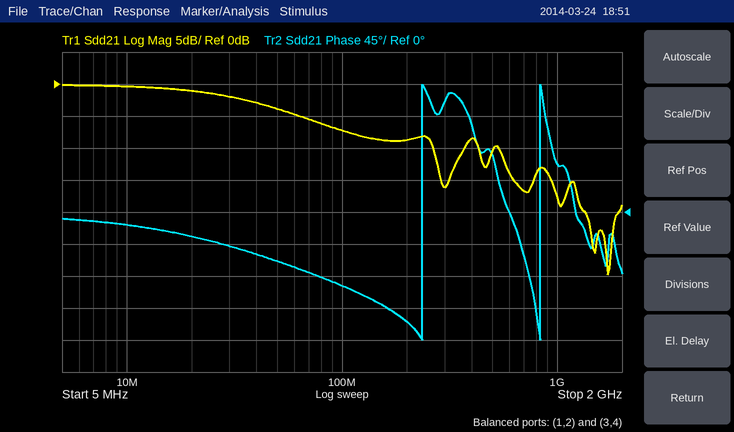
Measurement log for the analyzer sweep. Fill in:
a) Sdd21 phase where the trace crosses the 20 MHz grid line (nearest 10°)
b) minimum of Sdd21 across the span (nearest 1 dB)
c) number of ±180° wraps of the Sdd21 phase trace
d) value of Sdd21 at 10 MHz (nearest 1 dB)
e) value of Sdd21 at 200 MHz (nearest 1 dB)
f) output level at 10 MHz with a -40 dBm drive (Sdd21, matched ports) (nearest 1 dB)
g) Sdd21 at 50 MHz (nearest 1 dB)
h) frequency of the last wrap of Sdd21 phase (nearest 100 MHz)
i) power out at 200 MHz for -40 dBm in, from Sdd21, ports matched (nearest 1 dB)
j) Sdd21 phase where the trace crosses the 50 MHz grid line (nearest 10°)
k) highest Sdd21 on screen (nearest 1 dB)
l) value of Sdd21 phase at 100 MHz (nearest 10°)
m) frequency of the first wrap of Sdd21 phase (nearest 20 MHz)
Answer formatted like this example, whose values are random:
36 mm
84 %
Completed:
-30°
-30 dB
2
0 dB
-9 dB
-40 dBm
-4 dB
800 MHz
-49 dBm
-70°
0 dB
-100°
240 MHz
